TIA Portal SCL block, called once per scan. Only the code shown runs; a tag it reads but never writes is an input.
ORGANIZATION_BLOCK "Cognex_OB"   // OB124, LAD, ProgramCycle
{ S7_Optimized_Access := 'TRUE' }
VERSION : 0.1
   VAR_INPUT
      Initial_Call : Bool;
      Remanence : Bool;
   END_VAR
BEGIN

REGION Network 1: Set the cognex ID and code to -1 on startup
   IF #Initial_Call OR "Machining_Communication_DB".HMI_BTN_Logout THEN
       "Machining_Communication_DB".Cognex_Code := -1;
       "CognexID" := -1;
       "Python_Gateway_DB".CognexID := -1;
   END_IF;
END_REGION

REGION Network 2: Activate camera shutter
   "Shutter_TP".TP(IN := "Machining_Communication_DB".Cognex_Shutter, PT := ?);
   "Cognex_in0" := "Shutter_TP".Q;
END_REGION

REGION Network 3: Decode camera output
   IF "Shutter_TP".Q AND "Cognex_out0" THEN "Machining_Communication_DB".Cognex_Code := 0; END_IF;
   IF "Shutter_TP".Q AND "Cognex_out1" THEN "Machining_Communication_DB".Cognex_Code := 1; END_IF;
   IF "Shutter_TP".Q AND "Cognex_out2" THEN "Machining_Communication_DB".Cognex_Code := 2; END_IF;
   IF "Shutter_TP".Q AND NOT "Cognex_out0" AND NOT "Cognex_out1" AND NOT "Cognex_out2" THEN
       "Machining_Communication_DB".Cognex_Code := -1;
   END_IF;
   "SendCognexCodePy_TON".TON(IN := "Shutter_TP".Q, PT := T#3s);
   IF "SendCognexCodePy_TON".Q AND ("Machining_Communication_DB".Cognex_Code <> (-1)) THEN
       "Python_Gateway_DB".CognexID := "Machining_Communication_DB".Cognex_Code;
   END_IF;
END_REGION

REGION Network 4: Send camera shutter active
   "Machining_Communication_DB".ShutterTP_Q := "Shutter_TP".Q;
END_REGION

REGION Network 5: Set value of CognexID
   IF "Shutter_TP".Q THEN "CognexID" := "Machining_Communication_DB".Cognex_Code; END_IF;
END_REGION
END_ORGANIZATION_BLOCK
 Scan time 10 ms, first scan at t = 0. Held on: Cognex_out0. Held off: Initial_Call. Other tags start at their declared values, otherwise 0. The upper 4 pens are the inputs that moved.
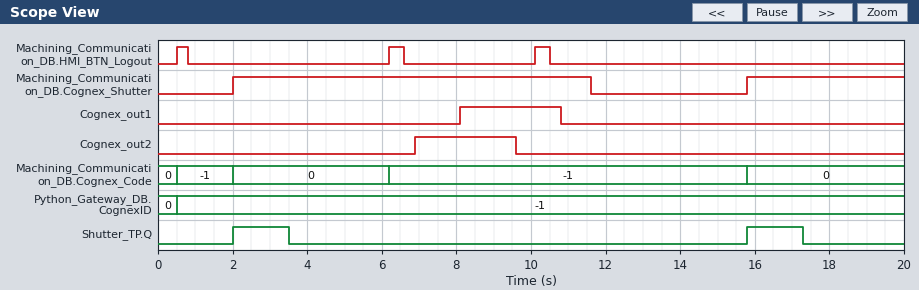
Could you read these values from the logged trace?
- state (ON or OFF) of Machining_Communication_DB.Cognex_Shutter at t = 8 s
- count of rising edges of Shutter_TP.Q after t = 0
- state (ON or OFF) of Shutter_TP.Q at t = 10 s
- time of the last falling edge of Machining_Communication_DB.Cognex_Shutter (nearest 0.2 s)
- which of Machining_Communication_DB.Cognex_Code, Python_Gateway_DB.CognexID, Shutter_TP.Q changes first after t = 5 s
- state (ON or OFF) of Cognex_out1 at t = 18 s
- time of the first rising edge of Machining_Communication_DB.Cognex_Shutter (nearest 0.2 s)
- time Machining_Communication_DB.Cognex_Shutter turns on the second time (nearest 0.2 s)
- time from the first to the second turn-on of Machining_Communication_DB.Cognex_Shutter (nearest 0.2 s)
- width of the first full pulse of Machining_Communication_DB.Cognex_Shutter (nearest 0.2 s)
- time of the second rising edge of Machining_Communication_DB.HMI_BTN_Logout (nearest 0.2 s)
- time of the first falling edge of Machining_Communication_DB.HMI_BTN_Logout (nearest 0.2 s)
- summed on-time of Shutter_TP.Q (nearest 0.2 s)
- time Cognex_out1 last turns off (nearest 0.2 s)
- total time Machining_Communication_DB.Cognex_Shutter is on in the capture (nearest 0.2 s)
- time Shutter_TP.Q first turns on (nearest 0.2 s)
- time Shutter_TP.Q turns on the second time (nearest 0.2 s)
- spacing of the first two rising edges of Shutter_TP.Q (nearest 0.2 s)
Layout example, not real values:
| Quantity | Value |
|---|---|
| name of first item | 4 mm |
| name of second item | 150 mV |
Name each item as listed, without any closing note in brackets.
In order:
| Quantity | Value |
|---|---|
| state (ON or OFF) of Machining_Communication_DB.Cognex_Shutter at t = 8 s | ON |
| count of rising edges of Shutter_TP.Q after t = 0 | 2 |
| state (ON or OFF) of Shutter_TP.Q at t = 10 s | OFF |
| time of the last falling edge of Machining_Communication_DB.Cognex_Shutter | 11.6 s |
| which of Machining_Communication_DB.Cognex_Code, Python_Gateway_DB.CognexID, Shutter_TP.Q changes first after t = 5 s | Machining_Communication_DB.Cognex_Code |
| state (ON or OFF) of Cognex_out1 at t = 18 s | OFF |
| time of the first rising edge of Machining_Communication_DB.Cognex_Shutter | 2.0 s |
| time Machining_Communication_DB.Cognex_Shutter turns on the second time | 15.8 s |
| time from the first to the second turn-on of Machining_Communication_DB.Cognex_Shutter | 13.8 s |
| width of the first full pulse of Machining_Communication_DB.Cognex_Shutter | 9.6 s |
| time of the second rising edge of Machining_Communication_DB.HMI_BTN_Logout | 6.2 s |
| time of the first falling edge of Machining_Communication_DB.HMI_BTN_Logout | 0.8 s |
| summed on-time of Shutter_TP.Q | 3.0 s |
| time Cognex_out1 last turns off | 10.8 s |
| total time Machining_Communication_DB.Cognex_Shutter is on in the capture | 13.8 s |
| time Shutter_TP.Q first turns on | 2.0 s |
| time Shutter_TP.Q turns on the second time | 15.8 s |
| spacing of the first two rising edges of Shutter_TP.Q | 13.8 s |
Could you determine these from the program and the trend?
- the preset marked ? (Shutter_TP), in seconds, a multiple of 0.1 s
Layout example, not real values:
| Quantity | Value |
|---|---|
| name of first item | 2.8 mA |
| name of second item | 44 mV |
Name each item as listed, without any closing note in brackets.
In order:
| Quantity | Value |
|---|---|
| the preset marked ? (Shutter_TP), in seconds, a multiple of 0.1 s | 1.5 s |
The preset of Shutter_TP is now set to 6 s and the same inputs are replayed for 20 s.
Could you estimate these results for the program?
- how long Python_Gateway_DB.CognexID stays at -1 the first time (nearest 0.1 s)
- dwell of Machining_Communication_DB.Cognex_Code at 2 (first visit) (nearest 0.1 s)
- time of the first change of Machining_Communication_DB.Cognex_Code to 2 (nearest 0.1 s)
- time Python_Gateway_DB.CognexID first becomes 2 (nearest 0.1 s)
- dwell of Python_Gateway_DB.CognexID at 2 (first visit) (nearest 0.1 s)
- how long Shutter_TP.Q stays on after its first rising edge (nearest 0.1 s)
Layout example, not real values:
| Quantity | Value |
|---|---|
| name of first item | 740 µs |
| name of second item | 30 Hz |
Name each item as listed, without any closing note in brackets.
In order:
| Quantity | Value |
|---|---|
| how long Python_Gateway_DB.CognexID stays at -1 the first time | 4.5 s |
| dwell of Machining_Communication_DB.Cognex_Code at 2 (first visit) | 3.2 s |
| time of the first change of Machining_Communication_DB.Cognex_Code to 2 | 6.9 s |
| time Python_Gateway_DB.CognexID first becomes 2 | 6.9 s |
| dwell of Python_Gateway_DB.CognexID at 2 (first visit) | 3.2 s |
| how long Shutter_TP.Q stays on after its first rising edge | 6.0 s |
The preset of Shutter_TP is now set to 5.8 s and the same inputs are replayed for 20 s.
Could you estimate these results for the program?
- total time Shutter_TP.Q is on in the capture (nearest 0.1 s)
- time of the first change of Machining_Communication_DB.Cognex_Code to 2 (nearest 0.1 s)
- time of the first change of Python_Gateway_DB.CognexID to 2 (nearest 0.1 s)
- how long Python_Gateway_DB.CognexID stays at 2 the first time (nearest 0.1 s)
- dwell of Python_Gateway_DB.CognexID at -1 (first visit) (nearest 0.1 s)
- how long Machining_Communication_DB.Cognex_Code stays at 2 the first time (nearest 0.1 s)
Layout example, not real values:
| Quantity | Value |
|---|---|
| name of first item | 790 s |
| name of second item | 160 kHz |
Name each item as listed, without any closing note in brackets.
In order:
| Quantity | Value |
|---|---|
| total time Shutter_TP.Q is on in the capture | 10.0 s |
| time of the first change of Machining_Communication_DB.Cognex_Code to 2 | 6.9 s |
| time of the first change of Python_Gateway_DB.CognexID to 2 | 6.9 s |
| how long Python_Gateway_DB.CognexID stays at 2 the first time | 3.2 s |
| dwell of Python_Gateway_DB.CognexID at -1 (first visit) | 4.5 s |
| how long Machining_Communication_DB.Cognex_Code stays at 2 the first time | 3.2 s |
